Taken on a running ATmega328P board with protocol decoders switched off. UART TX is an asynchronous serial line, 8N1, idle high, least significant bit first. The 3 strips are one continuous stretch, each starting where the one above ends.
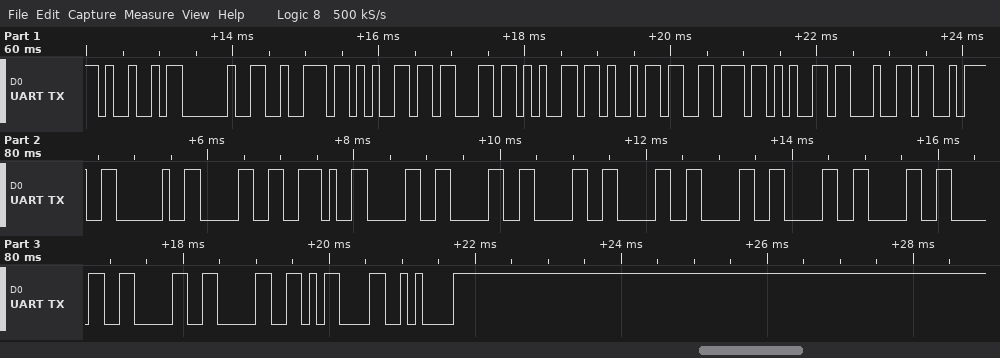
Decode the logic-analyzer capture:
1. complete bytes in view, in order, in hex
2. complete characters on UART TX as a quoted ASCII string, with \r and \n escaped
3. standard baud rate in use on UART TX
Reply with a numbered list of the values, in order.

1. 49 20 72 65 63 65 69 76 65 64 3A 20 30 2E 30 30 30 30 30 30 30 30 30 30 0D 0A
2. "I received: 0.0000000000\r\n"
3. 9600 baud
